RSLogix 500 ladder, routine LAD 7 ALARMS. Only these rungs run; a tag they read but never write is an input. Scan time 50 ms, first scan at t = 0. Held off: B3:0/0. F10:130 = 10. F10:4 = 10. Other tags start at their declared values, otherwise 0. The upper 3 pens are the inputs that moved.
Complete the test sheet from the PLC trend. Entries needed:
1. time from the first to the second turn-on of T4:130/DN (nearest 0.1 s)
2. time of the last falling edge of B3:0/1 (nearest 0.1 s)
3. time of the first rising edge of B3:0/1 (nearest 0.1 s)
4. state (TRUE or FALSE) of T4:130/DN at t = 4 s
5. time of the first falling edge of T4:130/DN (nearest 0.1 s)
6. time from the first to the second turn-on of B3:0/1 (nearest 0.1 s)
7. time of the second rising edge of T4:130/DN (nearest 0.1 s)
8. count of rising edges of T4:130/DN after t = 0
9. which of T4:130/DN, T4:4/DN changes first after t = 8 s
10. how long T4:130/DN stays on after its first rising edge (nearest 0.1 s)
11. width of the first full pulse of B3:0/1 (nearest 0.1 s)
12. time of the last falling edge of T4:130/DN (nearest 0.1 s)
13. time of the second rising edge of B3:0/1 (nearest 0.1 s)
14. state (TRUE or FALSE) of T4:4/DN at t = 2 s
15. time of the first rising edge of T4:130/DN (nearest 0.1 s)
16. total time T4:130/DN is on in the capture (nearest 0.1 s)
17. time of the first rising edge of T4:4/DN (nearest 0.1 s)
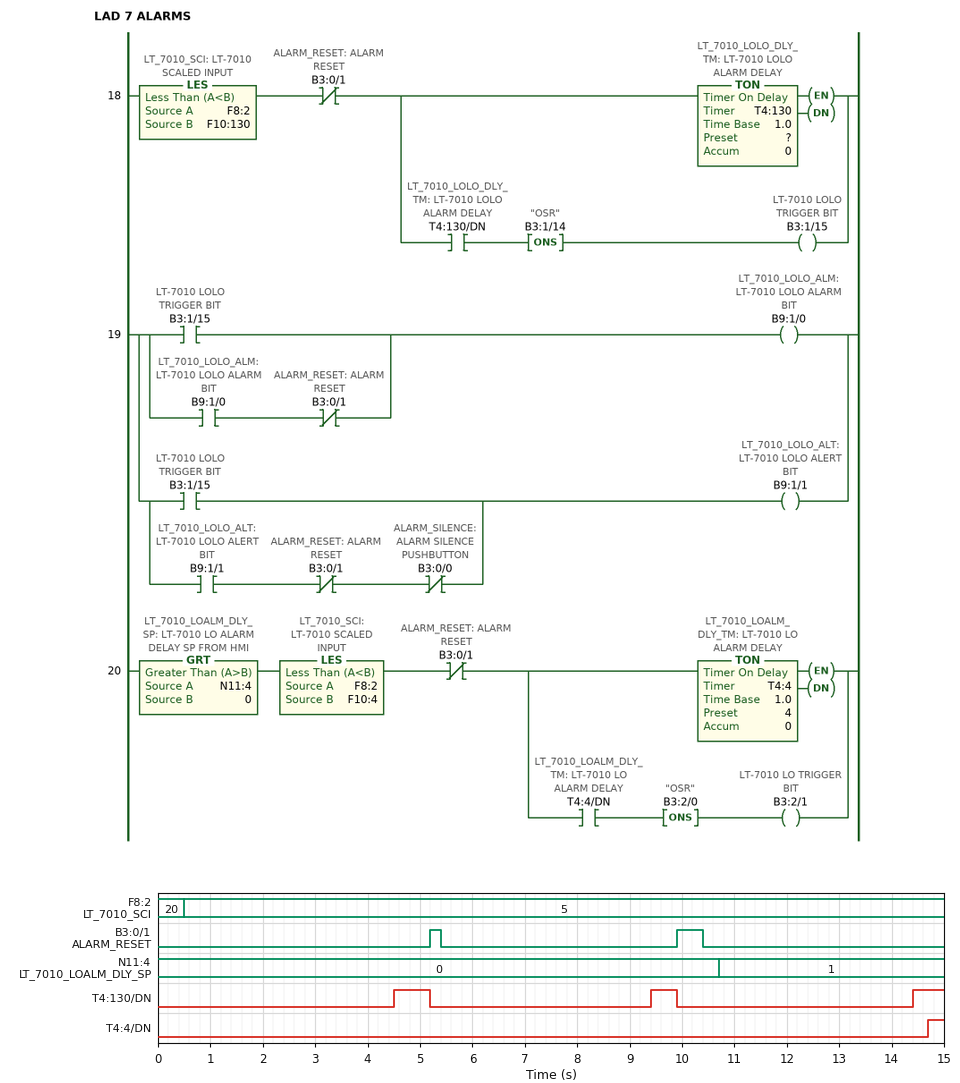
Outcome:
4.9 s
10.4 s
5.2 s
FALSE
5.2 s
4.7 s
9.4 s
3
T4:130/DN
0.7 s
0.2 s
9.9 s
9.9 s
FALSE
4.5 s
1.8 s
14.7 s
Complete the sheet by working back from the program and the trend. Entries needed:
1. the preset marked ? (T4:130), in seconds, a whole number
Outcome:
4 s
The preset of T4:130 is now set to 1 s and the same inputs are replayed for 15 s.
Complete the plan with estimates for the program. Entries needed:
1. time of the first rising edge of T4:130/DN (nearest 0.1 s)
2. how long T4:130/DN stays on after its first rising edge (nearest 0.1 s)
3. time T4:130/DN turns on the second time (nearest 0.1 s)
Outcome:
1.5 s
3.7 s
6.4 s
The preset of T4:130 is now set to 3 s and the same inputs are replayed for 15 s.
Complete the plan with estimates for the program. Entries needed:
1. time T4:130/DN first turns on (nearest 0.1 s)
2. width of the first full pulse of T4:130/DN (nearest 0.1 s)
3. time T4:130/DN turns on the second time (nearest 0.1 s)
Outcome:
3.5 s
1.7 s
8.4 s
